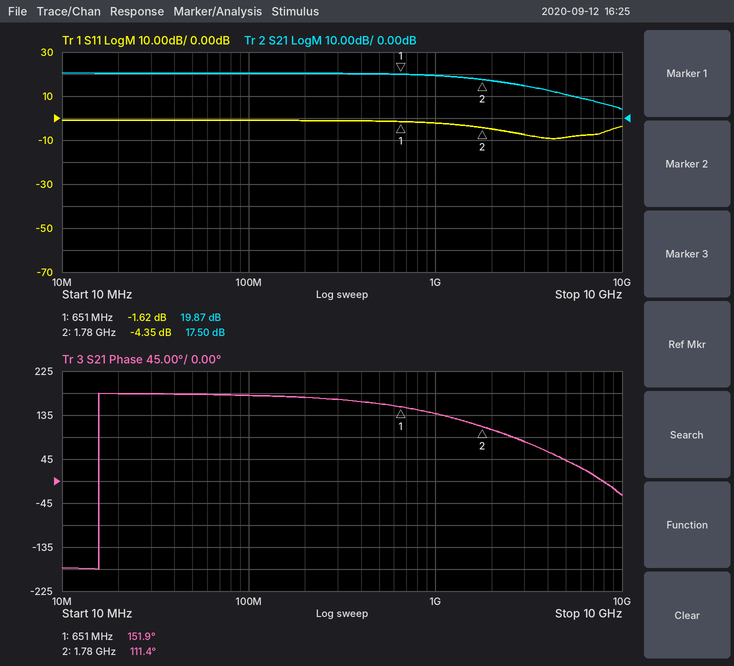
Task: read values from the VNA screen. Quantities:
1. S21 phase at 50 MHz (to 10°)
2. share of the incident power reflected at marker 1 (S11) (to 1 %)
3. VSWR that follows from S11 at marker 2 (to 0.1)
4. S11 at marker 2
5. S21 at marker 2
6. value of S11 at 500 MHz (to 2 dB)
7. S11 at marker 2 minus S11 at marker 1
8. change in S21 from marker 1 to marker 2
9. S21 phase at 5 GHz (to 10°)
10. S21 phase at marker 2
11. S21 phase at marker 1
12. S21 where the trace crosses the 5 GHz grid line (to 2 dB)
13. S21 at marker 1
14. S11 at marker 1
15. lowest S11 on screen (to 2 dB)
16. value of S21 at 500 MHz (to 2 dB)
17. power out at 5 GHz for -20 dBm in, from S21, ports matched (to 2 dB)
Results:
180°
69 %
4.1
-4.35 dB
17.50 dB
-2 dB
-2.73 dB
-2.37 dB
40°
111.4°
151.9°
10 dB
19.87 dB
-1.62 dB
-10 dB
20 dB
-10 dBm
